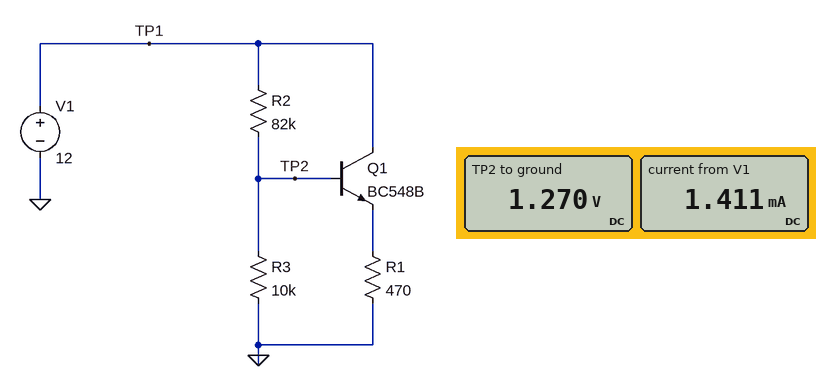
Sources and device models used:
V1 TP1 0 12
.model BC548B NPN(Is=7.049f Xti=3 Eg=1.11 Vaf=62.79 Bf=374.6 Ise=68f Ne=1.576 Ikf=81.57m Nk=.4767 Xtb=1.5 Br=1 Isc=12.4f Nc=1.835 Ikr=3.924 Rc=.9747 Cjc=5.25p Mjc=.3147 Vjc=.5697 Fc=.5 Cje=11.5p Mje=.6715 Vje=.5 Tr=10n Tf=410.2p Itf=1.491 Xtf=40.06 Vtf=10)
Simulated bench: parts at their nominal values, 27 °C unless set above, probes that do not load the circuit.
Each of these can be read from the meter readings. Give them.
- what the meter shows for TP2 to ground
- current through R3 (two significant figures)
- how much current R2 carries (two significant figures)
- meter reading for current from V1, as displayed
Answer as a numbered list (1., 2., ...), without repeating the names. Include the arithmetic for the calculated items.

1. 1.270 V
2. (1.27 V) / 10 kΩ = 130 µA
3. (12 V - 1.27 V) / 82 kΩ = 130 µA
4. 1.411 mA
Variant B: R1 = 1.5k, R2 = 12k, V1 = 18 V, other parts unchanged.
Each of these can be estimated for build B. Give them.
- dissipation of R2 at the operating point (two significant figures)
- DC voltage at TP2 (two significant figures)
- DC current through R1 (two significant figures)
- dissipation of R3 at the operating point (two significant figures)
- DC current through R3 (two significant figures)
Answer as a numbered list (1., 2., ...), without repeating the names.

1. 8.2 mW
2. 8.1 V
3. 4.9 mA
4. 6.6 mW
5. 810 µA
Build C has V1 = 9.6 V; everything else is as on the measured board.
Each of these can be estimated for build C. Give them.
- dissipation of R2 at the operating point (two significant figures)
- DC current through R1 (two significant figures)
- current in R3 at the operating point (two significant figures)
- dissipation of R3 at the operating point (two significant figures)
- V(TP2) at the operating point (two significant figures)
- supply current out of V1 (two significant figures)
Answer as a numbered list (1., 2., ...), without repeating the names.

1. 900 µW
2. 780 µA
3. 100 µA
4. 100 µW
5. 1.0 V
6. 880 µA
